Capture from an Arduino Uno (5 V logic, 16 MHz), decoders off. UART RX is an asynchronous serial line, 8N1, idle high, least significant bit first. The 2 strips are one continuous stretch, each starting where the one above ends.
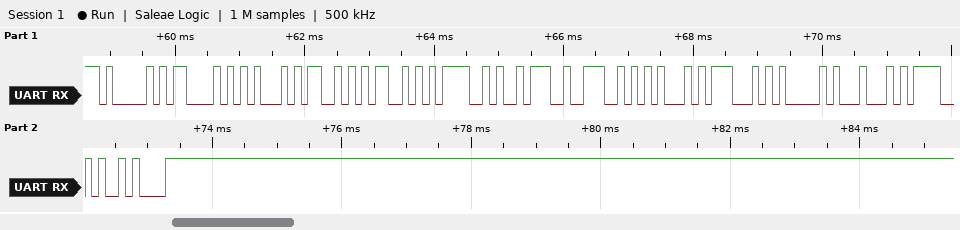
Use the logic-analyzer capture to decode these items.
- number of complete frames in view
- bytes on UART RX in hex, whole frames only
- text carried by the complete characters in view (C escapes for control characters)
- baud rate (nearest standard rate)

14
0x41 0x43 0x45 0x53 0x53 0x4F 0x3A 0x4E 0x45 0x47 0x41 0x44 0x4F 0x0A
"ACESSO:NEGADO\n"
9600 baud
